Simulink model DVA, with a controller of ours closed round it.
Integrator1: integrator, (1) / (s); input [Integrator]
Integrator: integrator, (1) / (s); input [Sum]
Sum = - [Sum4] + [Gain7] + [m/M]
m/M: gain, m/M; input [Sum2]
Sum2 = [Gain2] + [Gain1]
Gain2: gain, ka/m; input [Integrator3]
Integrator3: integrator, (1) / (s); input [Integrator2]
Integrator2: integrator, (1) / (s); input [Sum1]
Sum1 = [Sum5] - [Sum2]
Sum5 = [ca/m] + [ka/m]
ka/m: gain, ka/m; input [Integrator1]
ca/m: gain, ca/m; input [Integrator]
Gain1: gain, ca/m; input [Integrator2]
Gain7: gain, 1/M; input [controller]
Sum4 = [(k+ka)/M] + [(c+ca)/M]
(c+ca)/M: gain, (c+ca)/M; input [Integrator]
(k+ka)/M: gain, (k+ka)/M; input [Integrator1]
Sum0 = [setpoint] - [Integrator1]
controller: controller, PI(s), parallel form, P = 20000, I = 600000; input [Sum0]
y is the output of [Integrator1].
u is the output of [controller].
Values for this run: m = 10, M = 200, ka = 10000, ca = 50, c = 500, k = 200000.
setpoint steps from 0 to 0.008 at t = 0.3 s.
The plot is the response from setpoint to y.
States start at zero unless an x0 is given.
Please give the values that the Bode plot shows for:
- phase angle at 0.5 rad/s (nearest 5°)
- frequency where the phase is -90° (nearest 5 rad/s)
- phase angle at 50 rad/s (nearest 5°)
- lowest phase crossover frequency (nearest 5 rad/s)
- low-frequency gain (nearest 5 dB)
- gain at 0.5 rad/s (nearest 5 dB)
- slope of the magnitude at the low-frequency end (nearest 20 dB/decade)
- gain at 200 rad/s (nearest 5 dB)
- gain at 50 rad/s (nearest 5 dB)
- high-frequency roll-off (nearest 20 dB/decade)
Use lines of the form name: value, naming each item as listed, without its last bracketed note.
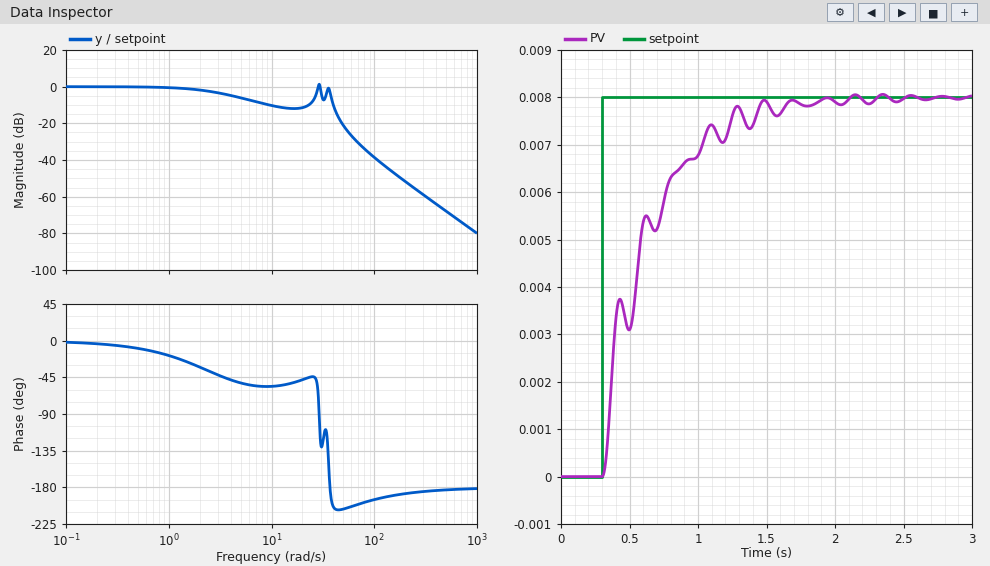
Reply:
phase angle at 0.5 rad/s: -10°
frequency where the phase is -90°: 30 rad/s
phase angle at 50 rad/s: -205°
lowest phase crossover frequency: 35 rad/s
low-frequency gain: 0 dB
gain at 0.5 rad/s: 0 dB
slope of the magnitude at the low-frequency end: 0 dB/decade
gain at 200 rad/s: -50 dB
gain at 50 rad/s: -20 dB
high-frequency roll-off: -40 dB/decade
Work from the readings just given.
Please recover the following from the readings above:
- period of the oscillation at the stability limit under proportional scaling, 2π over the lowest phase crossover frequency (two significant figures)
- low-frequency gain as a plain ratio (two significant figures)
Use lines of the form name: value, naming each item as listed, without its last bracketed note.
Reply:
period of the oscillation at the stability limit under proportional scaling, 2π over the lowest phase crossover frequency: 0.18 s
low-frequency gain as a plain ratio: 1.0
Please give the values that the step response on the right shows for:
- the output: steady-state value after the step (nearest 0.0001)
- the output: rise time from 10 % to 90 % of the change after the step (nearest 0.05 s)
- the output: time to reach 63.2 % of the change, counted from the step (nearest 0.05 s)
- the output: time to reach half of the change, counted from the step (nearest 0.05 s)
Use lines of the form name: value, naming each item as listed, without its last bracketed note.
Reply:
the output: steady-state value after the step: 0.0080
the output: rise time from 10 % to 90 % of the change after the step: 0.70 s
the output: time to reach 63.2 % of the change, counted from the step: 0.30 s
the output: time to reach half of the change, counted from the step: 0.25 s
